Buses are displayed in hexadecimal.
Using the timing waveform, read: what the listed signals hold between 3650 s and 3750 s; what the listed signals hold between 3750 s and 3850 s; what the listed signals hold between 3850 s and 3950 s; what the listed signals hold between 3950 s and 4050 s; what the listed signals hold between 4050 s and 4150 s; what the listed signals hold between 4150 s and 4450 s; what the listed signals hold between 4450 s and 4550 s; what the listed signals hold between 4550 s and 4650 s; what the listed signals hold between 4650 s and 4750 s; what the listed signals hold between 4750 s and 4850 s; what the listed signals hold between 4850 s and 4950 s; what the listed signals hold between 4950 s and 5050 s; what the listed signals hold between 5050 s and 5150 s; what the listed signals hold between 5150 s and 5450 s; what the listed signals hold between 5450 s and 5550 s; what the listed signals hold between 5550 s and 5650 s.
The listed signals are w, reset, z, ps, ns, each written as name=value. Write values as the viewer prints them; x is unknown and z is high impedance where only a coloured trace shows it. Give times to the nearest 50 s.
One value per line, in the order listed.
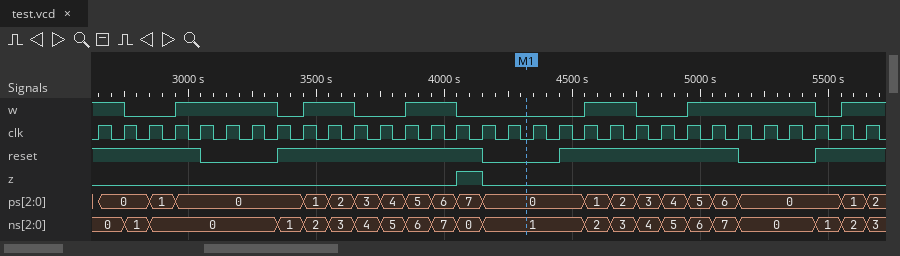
w=0, reset=1, z=0, ps=3, ns=4
w=0, reset=1, z=0, ps=4, ns=5
w=1, reset=1, z=0, ps=5, ns=6
w=1, reset=1, z=0, ps=6, ns=7
w=0, reset=1, z=1, ps=7, ns=0
w=0, reset=0, z=0, ps=0, ns=1
w=0, reset=1, z=0, ps=0, ns=1
w=1, reset=1, z=0, ps=1, ns=2
w=1, reset=1, z=0, ps=2, ns=3
w=0, reset=1, z=0, ps=3, ns=4
w=0, reset=1, z=0, ps=4, ns=5
w=1, reset=1, z=0, ps=5, ns=6
w=1, reset=1, z=0, ps=6, ns=7
w=1, reset=0, z=0, ps=0, ns=0
w=0, reset=1, z=0, ps=0, ns=1
w=1, reset=1, z=0, ps=1, ns=2
